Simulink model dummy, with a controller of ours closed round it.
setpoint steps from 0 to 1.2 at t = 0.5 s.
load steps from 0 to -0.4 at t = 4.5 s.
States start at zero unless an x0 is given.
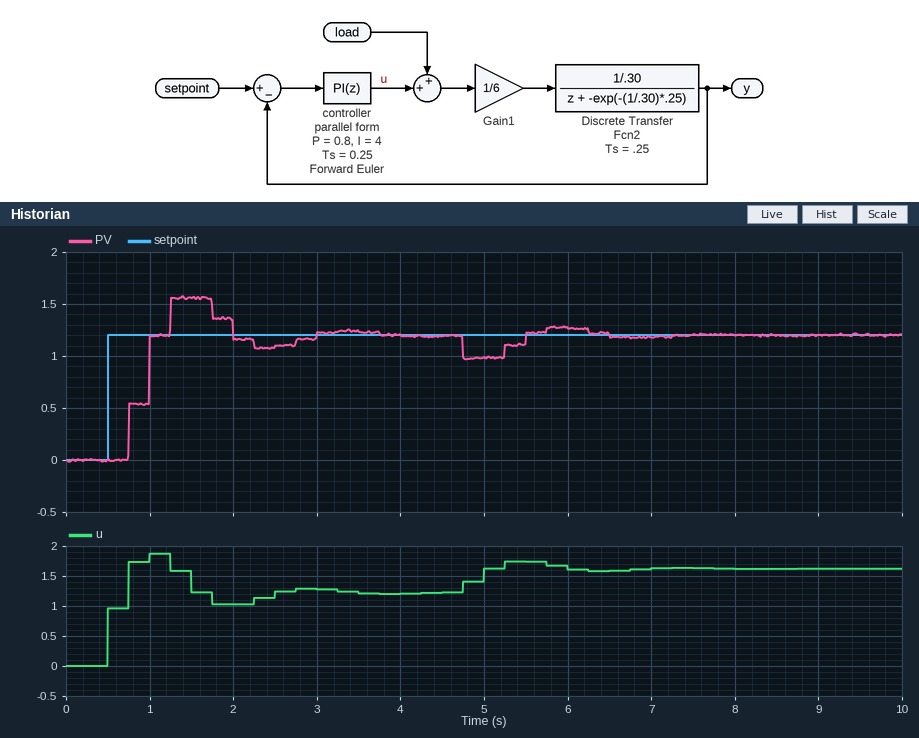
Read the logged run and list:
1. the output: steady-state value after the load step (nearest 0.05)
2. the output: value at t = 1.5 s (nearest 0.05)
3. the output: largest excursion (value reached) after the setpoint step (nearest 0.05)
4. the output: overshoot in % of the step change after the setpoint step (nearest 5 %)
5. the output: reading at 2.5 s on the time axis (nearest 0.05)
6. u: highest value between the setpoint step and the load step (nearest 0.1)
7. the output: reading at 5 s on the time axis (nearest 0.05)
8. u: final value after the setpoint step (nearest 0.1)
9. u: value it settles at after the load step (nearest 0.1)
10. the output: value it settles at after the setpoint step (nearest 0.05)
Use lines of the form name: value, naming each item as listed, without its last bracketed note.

the output: steady-state value after the load step: 1.20
the output: value at t = 1.5 s: 1.55
the output: largest excursion (value reached) after the setpoint step: 1.55
the output: overshoot in % of the step change after the setpoint step: 30 %
the output: reading at 2.5 s on the time axis: 1.10
u: highest value between the setpoint step and the load step: 1.9
the output: reading at 5 s on the time axis: 1.00
u: final value after the setpoint step: 1.2
u: value it settles at after the load step: 1.6
the output: value it settles at after the setpoint step: 1.20
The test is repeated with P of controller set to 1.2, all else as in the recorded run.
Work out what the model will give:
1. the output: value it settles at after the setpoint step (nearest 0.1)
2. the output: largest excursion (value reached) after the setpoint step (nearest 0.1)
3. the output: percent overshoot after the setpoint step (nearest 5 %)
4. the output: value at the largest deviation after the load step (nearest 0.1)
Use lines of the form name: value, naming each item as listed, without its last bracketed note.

the output: value it settles at after the setpoint step: 1.2
the output: largest excursion (value reached) after the setpoint step: 1.4
the output: percent overshoot after the setpoint step: 15 %
the output: value at the largest deviation after the load step: 1.0
